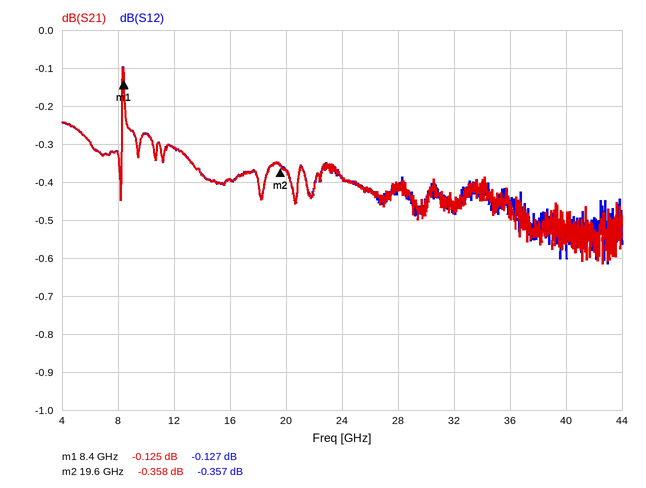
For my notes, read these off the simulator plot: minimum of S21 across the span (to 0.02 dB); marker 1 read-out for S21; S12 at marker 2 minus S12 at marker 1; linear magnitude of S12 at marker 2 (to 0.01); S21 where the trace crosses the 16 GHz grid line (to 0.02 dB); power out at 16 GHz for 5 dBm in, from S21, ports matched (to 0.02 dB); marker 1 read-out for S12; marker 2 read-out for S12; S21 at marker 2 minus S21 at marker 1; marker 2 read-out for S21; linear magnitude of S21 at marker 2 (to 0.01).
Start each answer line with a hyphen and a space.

- -0.62 dB
- -0.125 dB
- -0.230 dB
- 0.96
- -0.40 dB
- 4.60 dBm
- -0.127 dB
- -0.357 dB
- -0.233 dB
- -0.358 dB
- 0.96
